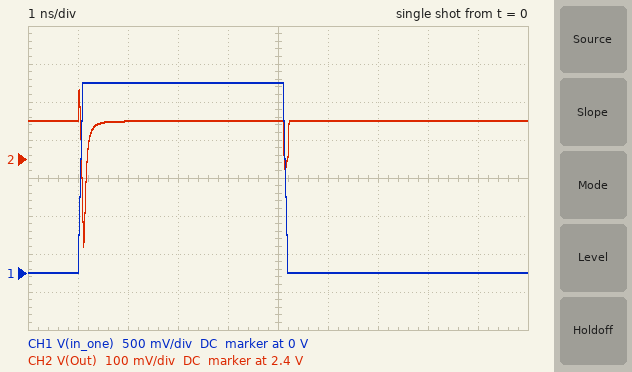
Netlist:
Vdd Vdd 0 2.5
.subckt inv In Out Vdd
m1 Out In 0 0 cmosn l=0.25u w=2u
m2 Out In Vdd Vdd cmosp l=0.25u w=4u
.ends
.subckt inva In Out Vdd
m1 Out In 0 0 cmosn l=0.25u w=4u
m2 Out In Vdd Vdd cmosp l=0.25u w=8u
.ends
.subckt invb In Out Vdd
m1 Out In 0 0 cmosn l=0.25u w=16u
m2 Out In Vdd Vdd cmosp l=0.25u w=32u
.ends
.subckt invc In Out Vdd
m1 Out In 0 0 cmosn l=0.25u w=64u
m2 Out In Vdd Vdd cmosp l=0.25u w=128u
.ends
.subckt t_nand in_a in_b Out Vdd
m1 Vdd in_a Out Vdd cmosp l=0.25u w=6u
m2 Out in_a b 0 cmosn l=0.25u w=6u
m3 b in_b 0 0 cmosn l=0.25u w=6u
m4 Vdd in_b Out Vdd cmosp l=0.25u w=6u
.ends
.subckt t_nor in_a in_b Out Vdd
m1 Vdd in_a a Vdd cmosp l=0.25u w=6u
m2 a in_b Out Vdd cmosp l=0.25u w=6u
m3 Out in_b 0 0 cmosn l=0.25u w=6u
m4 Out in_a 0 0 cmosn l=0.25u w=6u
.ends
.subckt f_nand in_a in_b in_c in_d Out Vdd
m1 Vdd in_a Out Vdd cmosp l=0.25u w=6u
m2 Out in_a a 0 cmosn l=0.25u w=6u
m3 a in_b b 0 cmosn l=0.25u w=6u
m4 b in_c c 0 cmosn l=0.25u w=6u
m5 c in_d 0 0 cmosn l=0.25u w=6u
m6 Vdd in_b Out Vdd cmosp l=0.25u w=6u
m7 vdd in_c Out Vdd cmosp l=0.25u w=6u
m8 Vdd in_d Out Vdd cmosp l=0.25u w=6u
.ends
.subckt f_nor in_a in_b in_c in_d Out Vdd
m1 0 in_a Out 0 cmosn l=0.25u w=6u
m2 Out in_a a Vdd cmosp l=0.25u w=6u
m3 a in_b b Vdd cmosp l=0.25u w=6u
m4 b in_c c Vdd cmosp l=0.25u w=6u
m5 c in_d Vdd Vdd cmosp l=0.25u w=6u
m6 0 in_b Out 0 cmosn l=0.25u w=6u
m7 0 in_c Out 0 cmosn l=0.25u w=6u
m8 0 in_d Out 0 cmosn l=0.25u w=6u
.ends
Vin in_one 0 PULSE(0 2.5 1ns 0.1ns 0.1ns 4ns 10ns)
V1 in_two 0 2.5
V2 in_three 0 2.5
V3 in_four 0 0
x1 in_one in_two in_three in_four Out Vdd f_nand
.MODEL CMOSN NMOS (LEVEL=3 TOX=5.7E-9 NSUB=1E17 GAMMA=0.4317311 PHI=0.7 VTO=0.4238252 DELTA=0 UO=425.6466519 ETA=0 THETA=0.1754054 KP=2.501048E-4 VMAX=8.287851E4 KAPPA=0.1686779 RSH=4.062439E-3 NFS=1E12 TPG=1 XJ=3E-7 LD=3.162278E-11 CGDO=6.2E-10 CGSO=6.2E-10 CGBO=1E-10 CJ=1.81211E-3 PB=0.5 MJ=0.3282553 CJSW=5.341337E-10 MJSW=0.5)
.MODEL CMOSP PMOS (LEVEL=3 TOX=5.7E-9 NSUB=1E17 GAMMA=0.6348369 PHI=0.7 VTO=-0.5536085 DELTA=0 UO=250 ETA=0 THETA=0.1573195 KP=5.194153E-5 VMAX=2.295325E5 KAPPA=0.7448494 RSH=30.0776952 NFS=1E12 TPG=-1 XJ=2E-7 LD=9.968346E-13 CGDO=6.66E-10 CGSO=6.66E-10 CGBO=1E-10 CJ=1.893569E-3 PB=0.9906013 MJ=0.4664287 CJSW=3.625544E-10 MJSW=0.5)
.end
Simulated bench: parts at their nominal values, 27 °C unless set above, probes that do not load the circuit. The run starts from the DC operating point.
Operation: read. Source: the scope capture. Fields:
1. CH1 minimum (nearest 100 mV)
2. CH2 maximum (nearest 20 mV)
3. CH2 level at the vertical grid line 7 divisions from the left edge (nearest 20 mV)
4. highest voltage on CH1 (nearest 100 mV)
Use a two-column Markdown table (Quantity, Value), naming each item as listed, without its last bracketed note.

| Quantity | Value |
|---|---|
| CH1 minimum | 0 V |
| CH2 maximum | 2.58 V |
| CH2 level at the vertical grid line 7 divisions from the left edge | 2.50 V |
| highest voltage on CH1 | 2.5 V |
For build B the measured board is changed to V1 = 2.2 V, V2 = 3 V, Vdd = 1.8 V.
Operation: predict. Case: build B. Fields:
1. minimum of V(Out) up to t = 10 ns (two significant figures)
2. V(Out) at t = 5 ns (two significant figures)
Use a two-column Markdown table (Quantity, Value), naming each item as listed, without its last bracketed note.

| Quantity | Value |
|---|---|
| minimum of V(Out) up to t = 10 ns | 1.5 V |
| V(Out) at t = 5 ns | 1.8 V |
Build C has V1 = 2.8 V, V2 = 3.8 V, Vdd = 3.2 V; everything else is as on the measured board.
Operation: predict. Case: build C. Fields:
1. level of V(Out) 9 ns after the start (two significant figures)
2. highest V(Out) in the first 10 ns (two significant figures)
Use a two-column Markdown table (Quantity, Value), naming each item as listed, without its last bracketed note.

| Quantity | Value |
|---|---|
| level of V(Out) 9 ns after the start | 3.2 V |
| highest V(Out) in the first 10 ns | 3.3 V |
